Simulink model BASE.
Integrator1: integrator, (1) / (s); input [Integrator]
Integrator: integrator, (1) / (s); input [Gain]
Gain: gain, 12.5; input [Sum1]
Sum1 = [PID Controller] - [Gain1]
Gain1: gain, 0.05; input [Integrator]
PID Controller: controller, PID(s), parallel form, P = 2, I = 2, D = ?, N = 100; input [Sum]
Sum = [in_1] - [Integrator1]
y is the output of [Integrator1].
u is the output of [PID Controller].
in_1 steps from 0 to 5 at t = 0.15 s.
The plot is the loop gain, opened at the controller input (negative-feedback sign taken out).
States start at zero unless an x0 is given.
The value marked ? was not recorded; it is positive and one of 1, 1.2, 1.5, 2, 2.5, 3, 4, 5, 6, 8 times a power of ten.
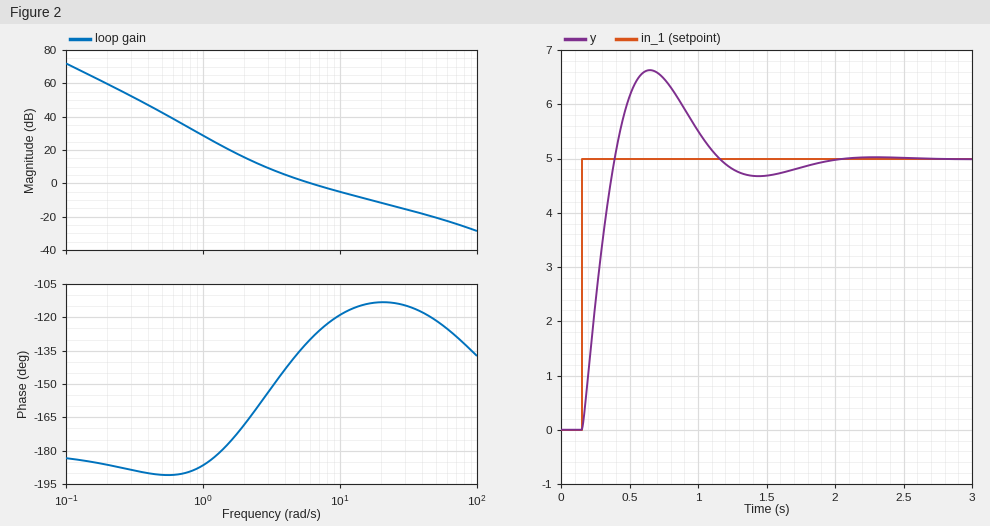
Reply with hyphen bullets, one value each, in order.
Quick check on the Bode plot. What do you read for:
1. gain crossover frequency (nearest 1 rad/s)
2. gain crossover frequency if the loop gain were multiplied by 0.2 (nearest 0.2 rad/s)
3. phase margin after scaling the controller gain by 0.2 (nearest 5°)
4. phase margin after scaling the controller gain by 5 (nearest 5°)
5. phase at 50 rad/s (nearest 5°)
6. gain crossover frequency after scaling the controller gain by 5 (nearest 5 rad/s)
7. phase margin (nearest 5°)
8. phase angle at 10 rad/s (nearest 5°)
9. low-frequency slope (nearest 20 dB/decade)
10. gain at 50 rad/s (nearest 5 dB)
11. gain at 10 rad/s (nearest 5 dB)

- 6 rad/s
- 2.2 rad/s
- 15°
- 65°
- -120°
- 25 rad/s
- 50°
- -120°
- -40 dB/decade
- -20 dB
- -5 dB
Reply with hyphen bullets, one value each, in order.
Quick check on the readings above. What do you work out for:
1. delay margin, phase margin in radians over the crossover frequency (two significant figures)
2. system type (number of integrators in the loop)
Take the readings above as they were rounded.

- 0.15 s
- 2
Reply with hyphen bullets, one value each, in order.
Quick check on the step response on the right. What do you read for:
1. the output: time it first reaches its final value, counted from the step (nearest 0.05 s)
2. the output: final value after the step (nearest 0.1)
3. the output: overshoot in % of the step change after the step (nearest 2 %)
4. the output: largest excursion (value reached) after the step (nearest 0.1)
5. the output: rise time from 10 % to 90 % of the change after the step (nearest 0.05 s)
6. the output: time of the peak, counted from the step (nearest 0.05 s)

- 0.25 s
- 5.0
- 32 %
- 6.6
- 0.20 s
- 0.50 s
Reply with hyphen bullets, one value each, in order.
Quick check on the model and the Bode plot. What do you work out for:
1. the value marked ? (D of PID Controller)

- 0.4
